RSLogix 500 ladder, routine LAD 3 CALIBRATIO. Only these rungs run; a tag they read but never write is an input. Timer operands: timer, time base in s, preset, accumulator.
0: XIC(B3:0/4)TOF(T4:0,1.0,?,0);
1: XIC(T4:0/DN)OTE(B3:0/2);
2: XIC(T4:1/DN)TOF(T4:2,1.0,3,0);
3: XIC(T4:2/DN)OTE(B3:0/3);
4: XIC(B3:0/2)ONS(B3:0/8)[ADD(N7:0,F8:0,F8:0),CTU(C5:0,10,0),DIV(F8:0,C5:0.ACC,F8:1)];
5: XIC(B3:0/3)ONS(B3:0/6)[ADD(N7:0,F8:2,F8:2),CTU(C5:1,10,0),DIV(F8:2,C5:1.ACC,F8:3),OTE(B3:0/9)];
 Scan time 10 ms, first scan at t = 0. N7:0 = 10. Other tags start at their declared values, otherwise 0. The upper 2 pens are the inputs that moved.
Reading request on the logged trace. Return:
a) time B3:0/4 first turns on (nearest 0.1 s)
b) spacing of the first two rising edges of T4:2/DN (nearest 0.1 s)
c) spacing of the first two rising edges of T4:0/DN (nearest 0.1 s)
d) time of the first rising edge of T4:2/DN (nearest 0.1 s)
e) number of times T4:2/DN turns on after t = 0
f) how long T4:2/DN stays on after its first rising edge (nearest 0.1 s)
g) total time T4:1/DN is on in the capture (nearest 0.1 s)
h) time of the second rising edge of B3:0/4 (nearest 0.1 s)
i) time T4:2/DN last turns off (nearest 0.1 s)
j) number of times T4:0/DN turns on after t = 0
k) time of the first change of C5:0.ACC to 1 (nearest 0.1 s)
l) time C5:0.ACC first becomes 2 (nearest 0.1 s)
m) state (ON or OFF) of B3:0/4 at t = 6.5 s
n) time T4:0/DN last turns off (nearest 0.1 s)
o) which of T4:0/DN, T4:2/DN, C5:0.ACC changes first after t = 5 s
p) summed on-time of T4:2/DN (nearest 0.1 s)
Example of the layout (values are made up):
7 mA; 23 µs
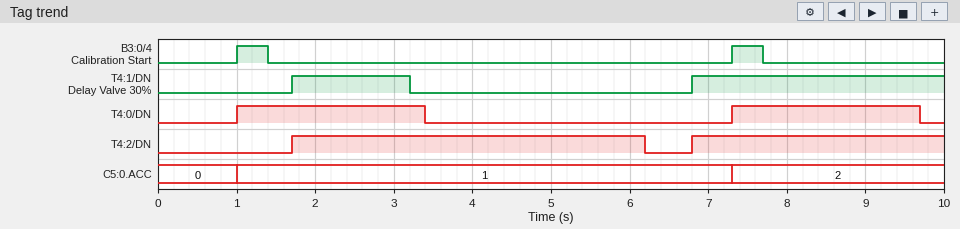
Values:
1.0 s; 5.1 s; 6.3 s; 1.7 s; 2; 4.5 s; 4.7 s; 7.3 s; 6.2 s; 2; 1.0 s; 7.3 s; OFF; 9.7 s; T4:2/DN; 7.7 s
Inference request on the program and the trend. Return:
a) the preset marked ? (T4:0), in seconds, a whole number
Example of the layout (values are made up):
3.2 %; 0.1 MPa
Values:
2 s
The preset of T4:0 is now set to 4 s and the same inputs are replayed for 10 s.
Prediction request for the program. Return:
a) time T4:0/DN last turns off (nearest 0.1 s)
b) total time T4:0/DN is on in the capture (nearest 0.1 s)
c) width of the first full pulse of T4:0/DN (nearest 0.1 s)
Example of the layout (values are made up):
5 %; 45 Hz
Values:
5.4 s; 7.1 s; 4.4 s
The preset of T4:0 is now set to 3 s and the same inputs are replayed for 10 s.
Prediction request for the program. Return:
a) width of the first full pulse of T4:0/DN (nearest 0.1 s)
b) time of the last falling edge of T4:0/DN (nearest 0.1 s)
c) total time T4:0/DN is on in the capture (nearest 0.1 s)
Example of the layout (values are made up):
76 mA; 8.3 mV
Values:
3.4 s; 4.4 s; 6.1 s
